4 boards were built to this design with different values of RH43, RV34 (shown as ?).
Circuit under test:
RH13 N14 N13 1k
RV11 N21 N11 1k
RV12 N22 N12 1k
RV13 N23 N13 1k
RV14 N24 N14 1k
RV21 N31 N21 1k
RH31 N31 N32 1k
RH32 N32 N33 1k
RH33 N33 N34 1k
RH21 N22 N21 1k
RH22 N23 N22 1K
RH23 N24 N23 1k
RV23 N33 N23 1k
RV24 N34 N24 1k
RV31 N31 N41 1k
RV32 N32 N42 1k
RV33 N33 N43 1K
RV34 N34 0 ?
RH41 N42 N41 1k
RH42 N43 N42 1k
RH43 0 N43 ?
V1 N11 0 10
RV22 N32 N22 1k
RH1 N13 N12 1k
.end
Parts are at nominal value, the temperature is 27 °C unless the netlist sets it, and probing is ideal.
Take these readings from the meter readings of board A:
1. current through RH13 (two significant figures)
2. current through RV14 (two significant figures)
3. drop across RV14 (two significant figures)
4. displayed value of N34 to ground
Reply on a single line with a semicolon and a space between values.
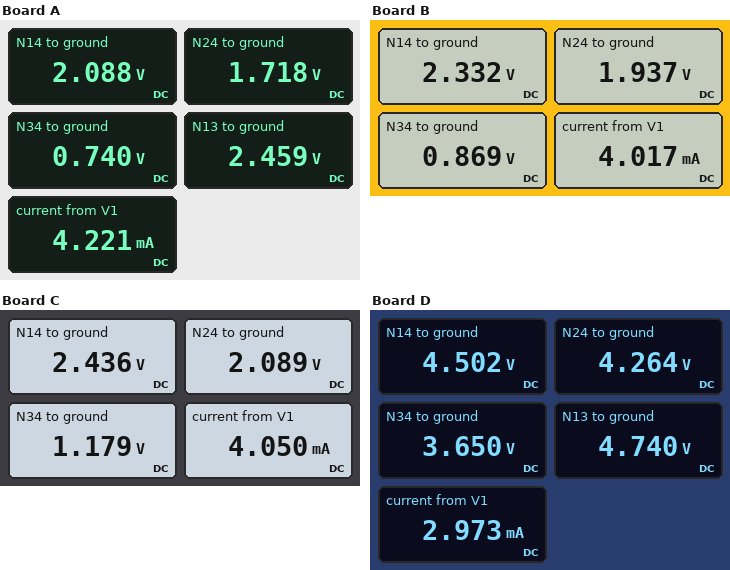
370 µA; 370 µA; 370 mV; 0.740 V
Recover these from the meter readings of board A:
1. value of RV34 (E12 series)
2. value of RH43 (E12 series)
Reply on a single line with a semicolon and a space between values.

390 Ω; 330 Ω
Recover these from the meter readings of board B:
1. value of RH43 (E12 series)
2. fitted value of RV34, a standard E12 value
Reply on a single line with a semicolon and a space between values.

820 Ω; 390 Ω
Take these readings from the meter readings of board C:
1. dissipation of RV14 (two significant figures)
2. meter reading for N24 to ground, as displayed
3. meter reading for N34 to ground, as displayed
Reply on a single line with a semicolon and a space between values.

120 µW; 2.089 V; 1.179 V
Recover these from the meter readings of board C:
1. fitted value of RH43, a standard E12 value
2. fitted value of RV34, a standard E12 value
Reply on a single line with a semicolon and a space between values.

470 Ω; 680 Ω
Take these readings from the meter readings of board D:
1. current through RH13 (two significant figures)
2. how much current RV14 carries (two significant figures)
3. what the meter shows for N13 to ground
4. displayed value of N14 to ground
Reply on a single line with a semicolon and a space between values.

240 µA; 240 µA; 4.740 V; 4.502 V
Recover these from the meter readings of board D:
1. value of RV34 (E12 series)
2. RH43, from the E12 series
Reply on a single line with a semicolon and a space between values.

3.3 kΩ; 1.8 kΩ
